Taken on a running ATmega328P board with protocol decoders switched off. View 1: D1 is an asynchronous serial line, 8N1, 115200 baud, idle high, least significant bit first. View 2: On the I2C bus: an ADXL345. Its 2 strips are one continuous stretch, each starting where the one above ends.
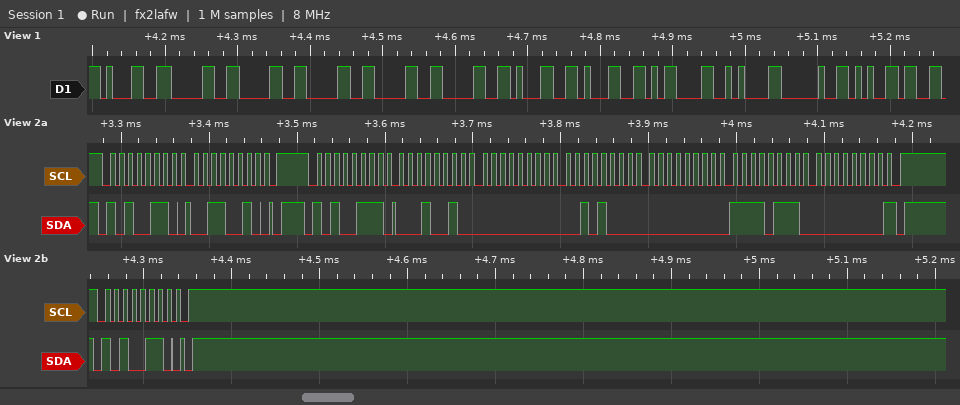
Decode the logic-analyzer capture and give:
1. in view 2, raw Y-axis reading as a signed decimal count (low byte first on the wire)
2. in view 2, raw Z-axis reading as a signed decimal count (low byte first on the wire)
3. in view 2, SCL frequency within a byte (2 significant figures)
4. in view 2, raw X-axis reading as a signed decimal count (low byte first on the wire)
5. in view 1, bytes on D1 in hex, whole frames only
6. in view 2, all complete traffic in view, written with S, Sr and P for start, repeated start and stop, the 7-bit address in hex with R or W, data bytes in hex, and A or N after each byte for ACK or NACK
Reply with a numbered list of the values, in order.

1. 40
2. 247
3. 100 kHz
4. 18
5. 31 30 30 30 30 30 31 31 0D 0A 20 65
6. S 53W A 32 A P S 53R A 12 A 00 A 28 A 00 A F7 A 00 N P S 53W A P
